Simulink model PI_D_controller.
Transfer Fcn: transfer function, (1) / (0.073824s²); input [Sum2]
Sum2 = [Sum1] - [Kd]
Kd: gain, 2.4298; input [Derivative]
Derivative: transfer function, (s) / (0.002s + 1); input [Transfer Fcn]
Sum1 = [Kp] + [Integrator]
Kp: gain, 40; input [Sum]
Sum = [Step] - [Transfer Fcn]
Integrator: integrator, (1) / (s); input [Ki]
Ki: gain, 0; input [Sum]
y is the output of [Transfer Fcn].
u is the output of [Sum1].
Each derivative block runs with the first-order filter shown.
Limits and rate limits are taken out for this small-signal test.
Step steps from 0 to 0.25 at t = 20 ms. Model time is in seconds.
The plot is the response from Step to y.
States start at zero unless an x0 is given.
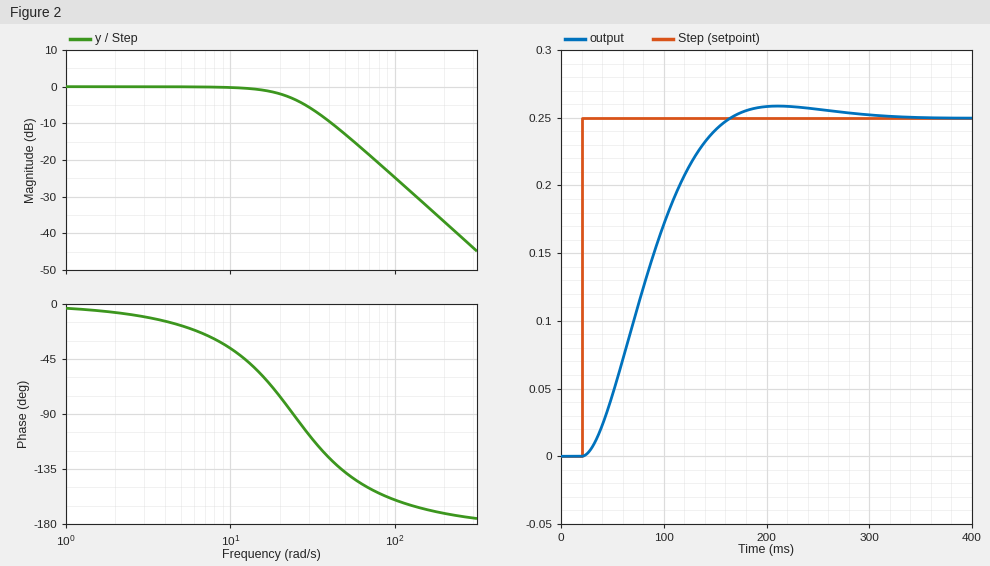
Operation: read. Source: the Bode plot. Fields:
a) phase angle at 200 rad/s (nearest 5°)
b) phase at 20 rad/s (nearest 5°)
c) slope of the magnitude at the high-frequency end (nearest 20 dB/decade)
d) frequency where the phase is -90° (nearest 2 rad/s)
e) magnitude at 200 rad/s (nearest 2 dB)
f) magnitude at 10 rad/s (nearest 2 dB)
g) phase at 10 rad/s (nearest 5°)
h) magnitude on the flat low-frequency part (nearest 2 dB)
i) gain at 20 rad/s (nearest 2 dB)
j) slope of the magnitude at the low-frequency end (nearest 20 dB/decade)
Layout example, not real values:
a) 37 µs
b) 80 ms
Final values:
a) -170°
b) -75°
c) -40 dB/decade
d) 24 rad/s
e) -36 dB
f) 0 dB
g) -35°
h) 0 dB
i) -2 dB
j) 0 dB/decade
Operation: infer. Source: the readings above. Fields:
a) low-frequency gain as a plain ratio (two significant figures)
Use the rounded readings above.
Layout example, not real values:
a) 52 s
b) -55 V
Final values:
a) 1.0
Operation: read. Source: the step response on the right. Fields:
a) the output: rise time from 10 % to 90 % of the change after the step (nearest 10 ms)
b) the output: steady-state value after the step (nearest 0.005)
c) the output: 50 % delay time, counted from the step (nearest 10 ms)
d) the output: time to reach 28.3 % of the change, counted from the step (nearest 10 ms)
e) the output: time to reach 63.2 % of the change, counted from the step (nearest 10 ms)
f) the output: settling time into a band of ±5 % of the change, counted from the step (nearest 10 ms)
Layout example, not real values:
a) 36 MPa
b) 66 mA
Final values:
a) 90 ms
b) 0.250
c) 60 ms
d) 40 ms
e) 70 ms
f) 130 ms
